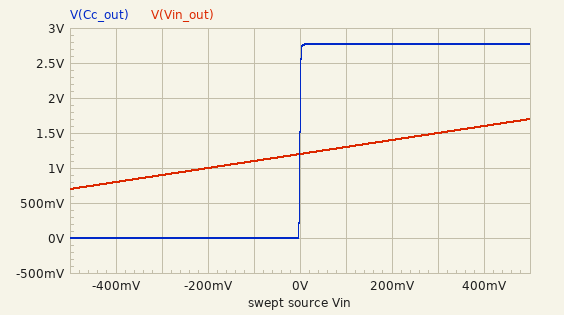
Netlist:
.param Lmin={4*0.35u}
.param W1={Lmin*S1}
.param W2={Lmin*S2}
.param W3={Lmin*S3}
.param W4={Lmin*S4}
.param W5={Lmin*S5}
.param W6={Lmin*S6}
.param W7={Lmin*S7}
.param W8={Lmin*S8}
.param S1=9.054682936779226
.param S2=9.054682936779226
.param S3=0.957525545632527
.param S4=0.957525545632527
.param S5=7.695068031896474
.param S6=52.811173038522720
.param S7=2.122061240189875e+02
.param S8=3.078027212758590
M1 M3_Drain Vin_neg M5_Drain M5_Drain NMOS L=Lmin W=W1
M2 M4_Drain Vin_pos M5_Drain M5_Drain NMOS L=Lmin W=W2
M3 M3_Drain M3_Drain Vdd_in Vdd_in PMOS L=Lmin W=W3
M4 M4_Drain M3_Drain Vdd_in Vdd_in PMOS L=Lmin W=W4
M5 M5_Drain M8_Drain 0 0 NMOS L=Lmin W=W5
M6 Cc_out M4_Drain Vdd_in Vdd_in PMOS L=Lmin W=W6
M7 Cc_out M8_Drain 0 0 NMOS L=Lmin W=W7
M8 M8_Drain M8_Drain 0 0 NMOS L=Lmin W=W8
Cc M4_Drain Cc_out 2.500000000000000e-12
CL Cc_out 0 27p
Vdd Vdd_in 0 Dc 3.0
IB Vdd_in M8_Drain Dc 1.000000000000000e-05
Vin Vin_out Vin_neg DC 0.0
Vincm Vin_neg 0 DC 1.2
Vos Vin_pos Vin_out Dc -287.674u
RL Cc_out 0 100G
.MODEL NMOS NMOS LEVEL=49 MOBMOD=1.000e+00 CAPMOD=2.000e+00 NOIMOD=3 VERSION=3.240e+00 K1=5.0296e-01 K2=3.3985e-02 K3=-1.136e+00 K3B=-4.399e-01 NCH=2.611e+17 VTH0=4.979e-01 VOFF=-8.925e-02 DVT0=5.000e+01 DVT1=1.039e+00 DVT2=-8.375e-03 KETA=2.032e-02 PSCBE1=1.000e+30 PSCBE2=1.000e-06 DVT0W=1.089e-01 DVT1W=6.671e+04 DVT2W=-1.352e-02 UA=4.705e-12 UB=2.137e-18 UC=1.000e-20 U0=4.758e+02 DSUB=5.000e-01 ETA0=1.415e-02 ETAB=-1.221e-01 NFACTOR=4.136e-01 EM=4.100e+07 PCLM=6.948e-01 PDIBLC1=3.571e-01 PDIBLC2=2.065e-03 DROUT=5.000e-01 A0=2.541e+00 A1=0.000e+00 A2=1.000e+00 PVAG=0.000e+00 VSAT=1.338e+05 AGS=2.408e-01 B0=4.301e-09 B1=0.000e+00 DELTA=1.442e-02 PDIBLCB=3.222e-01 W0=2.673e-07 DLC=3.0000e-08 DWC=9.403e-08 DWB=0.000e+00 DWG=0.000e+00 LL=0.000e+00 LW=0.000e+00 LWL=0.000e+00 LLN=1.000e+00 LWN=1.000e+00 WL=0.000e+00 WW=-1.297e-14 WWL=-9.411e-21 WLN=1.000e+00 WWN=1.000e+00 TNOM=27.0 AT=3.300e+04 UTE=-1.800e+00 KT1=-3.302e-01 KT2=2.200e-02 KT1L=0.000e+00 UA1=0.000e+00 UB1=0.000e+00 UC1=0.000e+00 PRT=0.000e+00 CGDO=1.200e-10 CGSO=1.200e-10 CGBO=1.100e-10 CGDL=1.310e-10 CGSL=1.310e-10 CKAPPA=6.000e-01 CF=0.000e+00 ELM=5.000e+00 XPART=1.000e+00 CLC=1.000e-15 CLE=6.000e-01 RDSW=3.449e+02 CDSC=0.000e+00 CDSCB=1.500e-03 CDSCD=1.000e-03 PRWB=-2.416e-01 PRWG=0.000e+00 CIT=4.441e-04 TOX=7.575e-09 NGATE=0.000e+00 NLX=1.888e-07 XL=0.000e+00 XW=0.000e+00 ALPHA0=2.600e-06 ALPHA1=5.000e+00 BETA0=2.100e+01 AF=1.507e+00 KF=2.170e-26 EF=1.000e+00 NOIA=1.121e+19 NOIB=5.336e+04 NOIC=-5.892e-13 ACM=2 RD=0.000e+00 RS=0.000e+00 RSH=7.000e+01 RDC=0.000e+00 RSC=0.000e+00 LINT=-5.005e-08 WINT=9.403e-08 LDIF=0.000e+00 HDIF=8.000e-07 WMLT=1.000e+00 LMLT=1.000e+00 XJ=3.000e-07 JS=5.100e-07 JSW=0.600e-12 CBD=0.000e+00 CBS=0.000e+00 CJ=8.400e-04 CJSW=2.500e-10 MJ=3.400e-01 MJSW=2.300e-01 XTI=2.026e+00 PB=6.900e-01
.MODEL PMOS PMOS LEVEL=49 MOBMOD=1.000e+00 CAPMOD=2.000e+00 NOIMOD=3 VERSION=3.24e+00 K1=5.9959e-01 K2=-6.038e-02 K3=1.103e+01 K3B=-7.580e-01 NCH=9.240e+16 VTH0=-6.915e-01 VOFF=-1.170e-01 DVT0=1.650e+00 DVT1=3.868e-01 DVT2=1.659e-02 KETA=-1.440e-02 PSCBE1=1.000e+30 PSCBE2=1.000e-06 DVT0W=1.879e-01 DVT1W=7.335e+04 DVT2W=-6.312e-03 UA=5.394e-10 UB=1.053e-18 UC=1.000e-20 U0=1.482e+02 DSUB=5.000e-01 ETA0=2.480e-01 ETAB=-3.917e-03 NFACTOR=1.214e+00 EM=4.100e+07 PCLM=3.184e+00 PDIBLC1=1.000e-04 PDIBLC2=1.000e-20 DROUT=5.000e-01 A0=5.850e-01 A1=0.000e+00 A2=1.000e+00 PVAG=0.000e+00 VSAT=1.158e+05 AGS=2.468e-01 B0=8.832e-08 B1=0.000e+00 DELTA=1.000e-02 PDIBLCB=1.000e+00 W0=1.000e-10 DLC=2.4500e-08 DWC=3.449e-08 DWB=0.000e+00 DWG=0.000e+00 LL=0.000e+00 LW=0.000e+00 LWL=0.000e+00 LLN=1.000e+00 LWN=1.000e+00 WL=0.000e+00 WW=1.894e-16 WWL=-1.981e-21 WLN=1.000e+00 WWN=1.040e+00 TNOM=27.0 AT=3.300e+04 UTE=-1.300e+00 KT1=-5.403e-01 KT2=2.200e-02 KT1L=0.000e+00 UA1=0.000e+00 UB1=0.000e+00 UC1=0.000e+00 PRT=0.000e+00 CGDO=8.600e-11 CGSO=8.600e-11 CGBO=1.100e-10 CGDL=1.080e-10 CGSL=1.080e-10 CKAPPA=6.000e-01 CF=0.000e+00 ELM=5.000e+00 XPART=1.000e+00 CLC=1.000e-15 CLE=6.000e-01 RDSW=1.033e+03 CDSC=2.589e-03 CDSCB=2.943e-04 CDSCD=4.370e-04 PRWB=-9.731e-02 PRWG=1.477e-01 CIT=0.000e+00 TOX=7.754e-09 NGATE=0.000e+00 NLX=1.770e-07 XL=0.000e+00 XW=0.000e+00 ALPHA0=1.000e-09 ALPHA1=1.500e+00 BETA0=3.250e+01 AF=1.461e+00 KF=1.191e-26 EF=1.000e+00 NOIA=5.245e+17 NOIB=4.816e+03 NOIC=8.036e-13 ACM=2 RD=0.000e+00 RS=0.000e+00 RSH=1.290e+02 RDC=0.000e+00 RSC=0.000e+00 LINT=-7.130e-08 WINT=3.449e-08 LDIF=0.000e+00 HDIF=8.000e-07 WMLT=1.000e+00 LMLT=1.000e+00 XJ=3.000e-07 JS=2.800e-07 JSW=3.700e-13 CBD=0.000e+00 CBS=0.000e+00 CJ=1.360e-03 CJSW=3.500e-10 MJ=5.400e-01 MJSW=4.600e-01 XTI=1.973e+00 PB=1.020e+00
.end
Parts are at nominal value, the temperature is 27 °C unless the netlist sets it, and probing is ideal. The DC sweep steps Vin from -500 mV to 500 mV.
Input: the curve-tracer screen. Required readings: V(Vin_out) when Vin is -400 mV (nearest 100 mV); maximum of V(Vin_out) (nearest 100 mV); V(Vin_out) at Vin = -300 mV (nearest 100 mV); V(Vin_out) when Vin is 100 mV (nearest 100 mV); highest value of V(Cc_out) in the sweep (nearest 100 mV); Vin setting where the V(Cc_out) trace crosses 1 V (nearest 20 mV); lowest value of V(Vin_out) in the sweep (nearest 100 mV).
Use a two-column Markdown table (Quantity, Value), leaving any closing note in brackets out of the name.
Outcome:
| Quantity | Value |
|---|---|
| V(Vin_out) when Vin is -400 mV | 800 mV |
| maximum of V(Vin_out) | 1.7 V |
| V(Vin_out) at Vin = -300 mV | 900 mV |
| V(Vin_out) when Vin is 100 mV | 1.3 V |
| highest value of V(Cc_out) in the sweep | 2.8 V |
| Vin setting where the V(Cc_out) trace crosses 1 V | 0 V |
| lowest value of V(Vin_out) in the sweep | 700 mV |
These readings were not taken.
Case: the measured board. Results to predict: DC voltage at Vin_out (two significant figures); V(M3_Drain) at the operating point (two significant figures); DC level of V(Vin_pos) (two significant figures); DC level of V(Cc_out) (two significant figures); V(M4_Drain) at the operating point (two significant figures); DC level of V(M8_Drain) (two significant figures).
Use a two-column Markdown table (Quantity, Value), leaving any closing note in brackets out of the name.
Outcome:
| Quantity | Value |
|---|---|
| DC voltage at Vin_out | 1.2 V |
| V(M3_Drain) at the operating point | 1.4 V |
| DC level of V(Vin_pos) | 1.2 V |
| DC level of V(Cc_out) | 1.5 V |
| V(M4_Drain) at the operating point | 1.5 V |
| DC level of V(M8_Drain) | 740 mV |
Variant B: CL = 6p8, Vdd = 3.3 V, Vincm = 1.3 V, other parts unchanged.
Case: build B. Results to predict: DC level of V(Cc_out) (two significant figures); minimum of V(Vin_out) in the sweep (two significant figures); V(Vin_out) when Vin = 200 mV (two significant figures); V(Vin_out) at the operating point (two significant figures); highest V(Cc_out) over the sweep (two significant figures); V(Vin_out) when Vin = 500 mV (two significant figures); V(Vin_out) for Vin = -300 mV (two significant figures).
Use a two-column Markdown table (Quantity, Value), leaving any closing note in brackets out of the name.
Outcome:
| Quantity | Value |
|---|---|
| DC level of V(Cc_out) | 1.7 V |
| minimum of V(Vin_out) in the sweep | 800 mV |
| V(Vin_out) when Vin = 200 mV | 1.5 V |
| V(Vin_out) at the operating point | 1.3 V |
| highest V(Cc_out) over the sweep | 3.1 V |
| V(Vin_out) when Vin = 500 mV | 1.8 V |
| V(Vin_out) for Vin = -300 mV | 1.0 V |
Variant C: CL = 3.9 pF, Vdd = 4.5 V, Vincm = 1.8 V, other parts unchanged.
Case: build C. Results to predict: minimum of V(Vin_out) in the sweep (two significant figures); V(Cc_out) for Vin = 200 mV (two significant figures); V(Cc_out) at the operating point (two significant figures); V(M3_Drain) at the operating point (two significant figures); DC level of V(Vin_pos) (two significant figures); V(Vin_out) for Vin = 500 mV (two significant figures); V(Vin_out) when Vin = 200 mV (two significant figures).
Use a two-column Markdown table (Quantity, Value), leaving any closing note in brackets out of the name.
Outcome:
| Quantity | Value |
|---|---|
| minimum of V(Vin_out) in the sweep | 1.3 V |
| V(Cc_out) for Vin = 200 mV | 4.3 V |
| V(Cc_out) at the operating point | 2.5 V |
| V(M3_Drain) at the operating point | 2.9 V |
| DC level of V(Vin_pos) | 1.8 V |
| V(Vin_out) for Vin = 500 mV | 2.3 V |
| V(Vin_out) when Vin = 200 mV | 2.0 V |
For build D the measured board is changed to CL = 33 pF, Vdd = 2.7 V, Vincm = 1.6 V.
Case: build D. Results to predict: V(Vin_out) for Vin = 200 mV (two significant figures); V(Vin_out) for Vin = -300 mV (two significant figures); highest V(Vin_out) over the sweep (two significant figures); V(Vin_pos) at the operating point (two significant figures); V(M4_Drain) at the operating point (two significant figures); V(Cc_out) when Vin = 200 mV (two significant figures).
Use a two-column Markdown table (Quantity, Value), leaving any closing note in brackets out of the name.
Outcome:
| Quantity | Value |
|---|---|
| V(Vin_out) for Vin = 200 mV | 1.8 V |
| V(Vin_out) for Vin = -300 mV | 1.3 V |
| highest V(Vin_out) over the sweep | 2.1 V |
| V(Vin_pos) at the operating point | 1.6 V |
| V(M4_Drain) at the operating point | 1.1 V |
| V(Cc_out) when Vin = 200 mV | 2.3 V |
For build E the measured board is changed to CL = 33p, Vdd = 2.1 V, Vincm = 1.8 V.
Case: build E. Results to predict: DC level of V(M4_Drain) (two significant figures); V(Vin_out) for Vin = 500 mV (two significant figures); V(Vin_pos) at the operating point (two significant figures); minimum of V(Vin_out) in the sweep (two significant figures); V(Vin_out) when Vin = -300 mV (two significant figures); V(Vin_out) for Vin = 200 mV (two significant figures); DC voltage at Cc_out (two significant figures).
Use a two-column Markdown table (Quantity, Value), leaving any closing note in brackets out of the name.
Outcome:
| Quantity | Value |
|---|---|
| DC level of V(M4_Drain) | 540 mV |
| V(Vin_out) for Vin = 500 mV | 2.3 V |
| V(Vin_pos) at the operating point | 1.8 V |
| minimum of V(Vin_out) in the sweep | 1.3 V |
| V(Vin_out) when Vin = -300 mV | 1.5 V |
| V(Vin_out) for Vin = 200 mV | 2.0 V |
| DC voltage at Cc_out | 1.5 V |
